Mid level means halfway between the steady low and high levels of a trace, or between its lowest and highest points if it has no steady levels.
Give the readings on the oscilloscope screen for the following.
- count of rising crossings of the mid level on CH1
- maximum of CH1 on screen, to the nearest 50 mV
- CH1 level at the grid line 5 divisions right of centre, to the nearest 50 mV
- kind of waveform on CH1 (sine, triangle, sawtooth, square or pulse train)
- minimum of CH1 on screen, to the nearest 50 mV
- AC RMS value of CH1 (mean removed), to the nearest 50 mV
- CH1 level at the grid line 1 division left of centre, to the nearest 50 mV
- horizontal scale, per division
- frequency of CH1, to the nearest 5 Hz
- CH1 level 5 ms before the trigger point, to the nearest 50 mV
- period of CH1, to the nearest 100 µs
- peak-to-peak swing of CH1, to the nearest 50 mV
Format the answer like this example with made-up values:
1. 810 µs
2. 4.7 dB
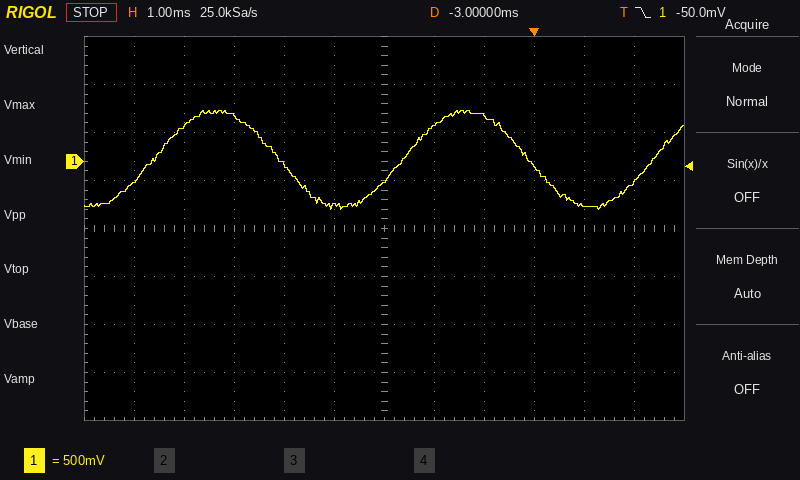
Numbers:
1. 3
2. 550 mV
3. -200 mV
4. sine
5. -500 mV
6. 350 mV
7. -450 mV
8. 1 ms
9. 200 Hz
10. -50 mV
11. 5.0 ms
12. 1.05 V
